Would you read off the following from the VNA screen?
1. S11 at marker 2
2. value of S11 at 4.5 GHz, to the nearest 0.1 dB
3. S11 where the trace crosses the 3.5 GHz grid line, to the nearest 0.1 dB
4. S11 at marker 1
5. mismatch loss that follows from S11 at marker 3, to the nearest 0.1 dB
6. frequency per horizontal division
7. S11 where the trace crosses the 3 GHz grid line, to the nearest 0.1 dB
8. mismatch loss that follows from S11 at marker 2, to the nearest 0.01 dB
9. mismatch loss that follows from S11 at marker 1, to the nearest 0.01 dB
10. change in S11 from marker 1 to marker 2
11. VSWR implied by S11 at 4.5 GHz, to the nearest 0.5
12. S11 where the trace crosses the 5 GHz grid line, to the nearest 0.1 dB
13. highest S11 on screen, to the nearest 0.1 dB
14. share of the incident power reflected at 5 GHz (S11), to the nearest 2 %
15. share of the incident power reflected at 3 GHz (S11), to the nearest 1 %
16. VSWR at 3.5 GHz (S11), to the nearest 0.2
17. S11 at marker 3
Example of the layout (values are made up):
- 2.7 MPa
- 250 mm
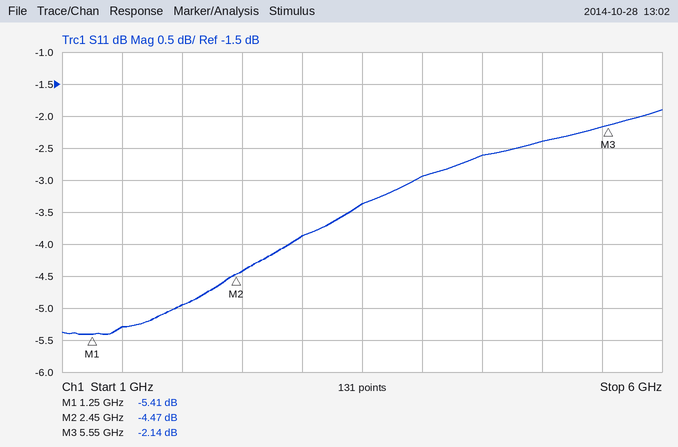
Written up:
- -4.47 dB
- -2.6 dB
- -3.4 dB
- -5.41 dB
- 4.1 dB
- 500 MHz
- -3.9 dB
- 1.92 dB
- 1.47 dB
- 0.94 dB
- 6.5
- -2.4 dB
- -1.9 dB
- 58 %
- 41 %
- 5.2
- -2.14 dB
